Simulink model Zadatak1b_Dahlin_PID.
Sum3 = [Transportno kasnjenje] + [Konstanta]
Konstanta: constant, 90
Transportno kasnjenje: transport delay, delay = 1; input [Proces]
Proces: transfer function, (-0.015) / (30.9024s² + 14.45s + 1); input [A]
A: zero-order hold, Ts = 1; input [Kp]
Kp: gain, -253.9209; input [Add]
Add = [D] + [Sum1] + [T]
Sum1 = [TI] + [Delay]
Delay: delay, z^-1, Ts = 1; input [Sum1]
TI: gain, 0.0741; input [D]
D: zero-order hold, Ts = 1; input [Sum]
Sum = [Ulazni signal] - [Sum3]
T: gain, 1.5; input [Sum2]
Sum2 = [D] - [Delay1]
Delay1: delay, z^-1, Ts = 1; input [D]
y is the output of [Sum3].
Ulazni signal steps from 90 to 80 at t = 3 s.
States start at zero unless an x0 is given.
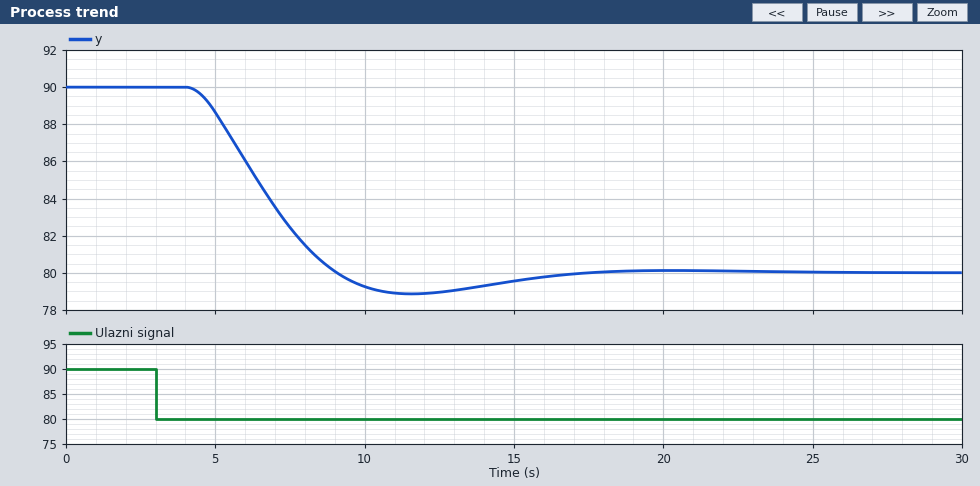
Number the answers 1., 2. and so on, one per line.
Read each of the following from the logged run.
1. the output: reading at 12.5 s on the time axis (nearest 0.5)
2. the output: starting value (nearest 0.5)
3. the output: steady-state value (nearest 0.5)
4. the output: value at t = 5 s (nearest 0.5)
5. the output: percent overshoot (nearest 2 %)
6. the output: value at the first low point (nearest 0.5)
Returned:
1. 79.0
2. 90.0
3. 80.0
4. 88.5
5. 12 %
6. 79.0
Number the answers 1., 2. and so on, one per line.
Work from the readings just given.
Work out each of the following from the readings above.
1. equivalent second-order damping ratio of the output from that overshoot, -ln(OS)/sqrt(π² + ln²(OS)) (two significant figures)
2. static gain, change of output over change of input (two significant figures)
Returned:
1. 0.56
2. 1.0
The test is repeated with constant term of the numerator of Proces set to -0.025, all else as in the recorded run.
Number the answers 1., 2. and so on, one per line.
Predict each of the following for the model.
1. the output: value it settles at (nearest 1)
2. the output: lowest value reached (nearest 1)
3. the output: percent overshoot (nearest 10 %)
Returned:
1. 80
2. 76
3. 40 %
